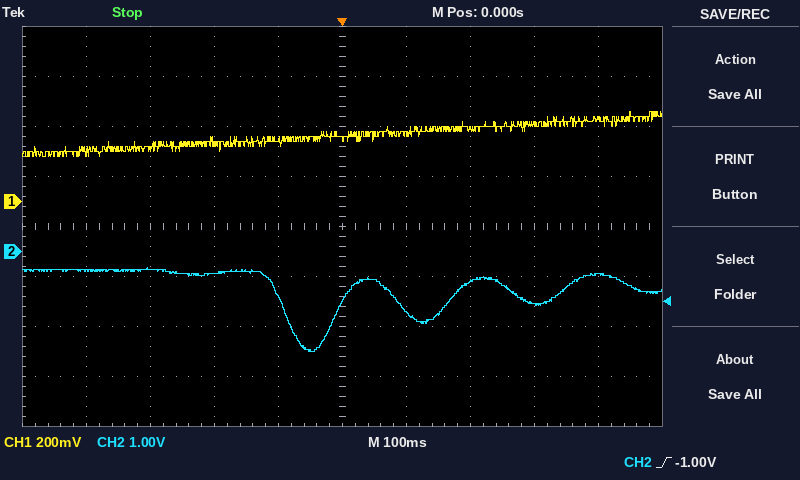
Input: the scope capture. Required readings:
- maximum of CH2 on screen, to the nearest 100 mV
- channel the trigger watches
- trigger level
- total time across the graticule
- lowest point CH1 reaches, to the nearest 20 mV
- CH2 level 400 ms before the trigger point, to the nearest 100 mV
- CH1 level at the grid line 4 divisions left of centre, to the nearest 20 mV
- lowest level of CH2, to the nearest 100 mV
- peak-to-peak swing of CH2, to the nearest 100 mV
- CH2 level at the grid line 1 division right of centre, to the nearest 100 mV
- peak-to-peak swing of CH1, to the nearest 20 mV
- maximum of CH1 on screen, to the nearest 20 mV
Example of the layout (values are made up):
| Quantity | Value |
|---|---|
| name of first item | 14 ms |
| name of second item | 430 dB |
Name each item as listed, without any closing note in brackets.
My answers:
| Quantity | Value |
|---|---|
| maximum of CH2 on screen, to the nearest 100 mV | -300 mV |
| channel the trigger watches | CH2 |
| trigger level | -1.00 V |
| total time across the graticule | 1 s |
| lowest point CH1 reaches, to the nearest 20 mV | 180 mV |
| CH2 level 400 ms before the trigger point, to the nearest 100 mV | -400 mV |
| CH1 level at the grid line 4 divisions left of centre, to the nearest 20 mV | 200 mV |
| lowest level of CH2, to the nearest 100 mV | -2.0 V |
| peak-to-peak swing of CH2, to the nearest 100 mV | 1.7 V |
| CH2 level at the grid line 1 division right of centre, to the nearest 100 mV | -1.2 V |
| peak-to-peak swing of CH1, to the nearest 20 mV | 180 mV |
| maximum of CH1 on screen, to the nearest 20 mV | 360 mV |
